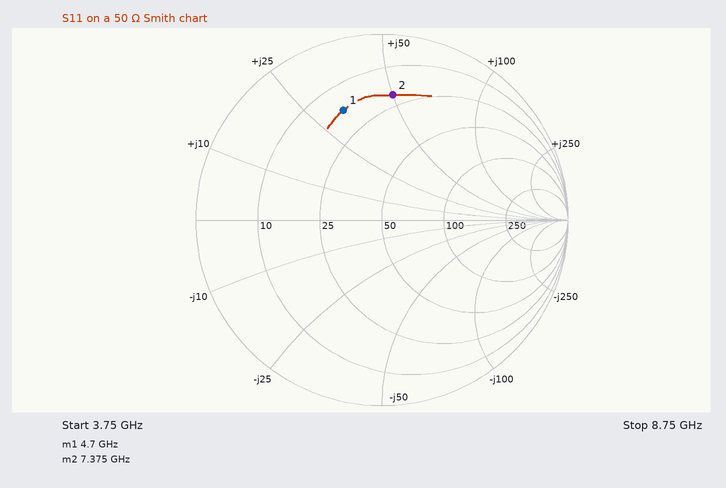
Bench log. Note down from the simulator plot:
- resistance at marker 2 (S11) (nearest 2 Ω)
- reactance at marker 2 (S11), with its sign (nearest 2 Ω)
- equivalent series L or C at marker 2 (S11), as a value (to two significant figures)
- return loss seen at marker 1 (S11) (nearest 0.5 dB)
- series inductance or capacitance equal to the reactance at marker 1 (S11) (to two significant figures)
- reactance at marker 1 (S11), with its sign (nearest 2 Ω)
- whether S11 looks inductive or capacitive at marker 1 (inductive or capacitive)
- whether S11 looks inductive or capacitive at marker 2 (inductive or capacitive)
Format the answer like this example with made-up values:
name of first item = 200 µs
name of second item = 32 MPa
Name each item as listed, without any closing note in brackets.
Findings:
resistance at marker 2 (S11) = 20 Ω
reactance at marker 2 (S11), with its sign = +50 Ω
equivalent series L or C at marker 2 (S11), as a value = 1.1 nH
return loss seen at marker 1 (S11) = 4.0 dB
series inductance or capacitance equal to the reactance at marker 1 (S11) = 1.1 nH
reactance at marker 1 (S11), with its sign = +32 Ω
whether S11 looks inductive or capacitive at marker 1 = inductive
whether S11 looks inductive or capacitive at marker 2 = inductive
